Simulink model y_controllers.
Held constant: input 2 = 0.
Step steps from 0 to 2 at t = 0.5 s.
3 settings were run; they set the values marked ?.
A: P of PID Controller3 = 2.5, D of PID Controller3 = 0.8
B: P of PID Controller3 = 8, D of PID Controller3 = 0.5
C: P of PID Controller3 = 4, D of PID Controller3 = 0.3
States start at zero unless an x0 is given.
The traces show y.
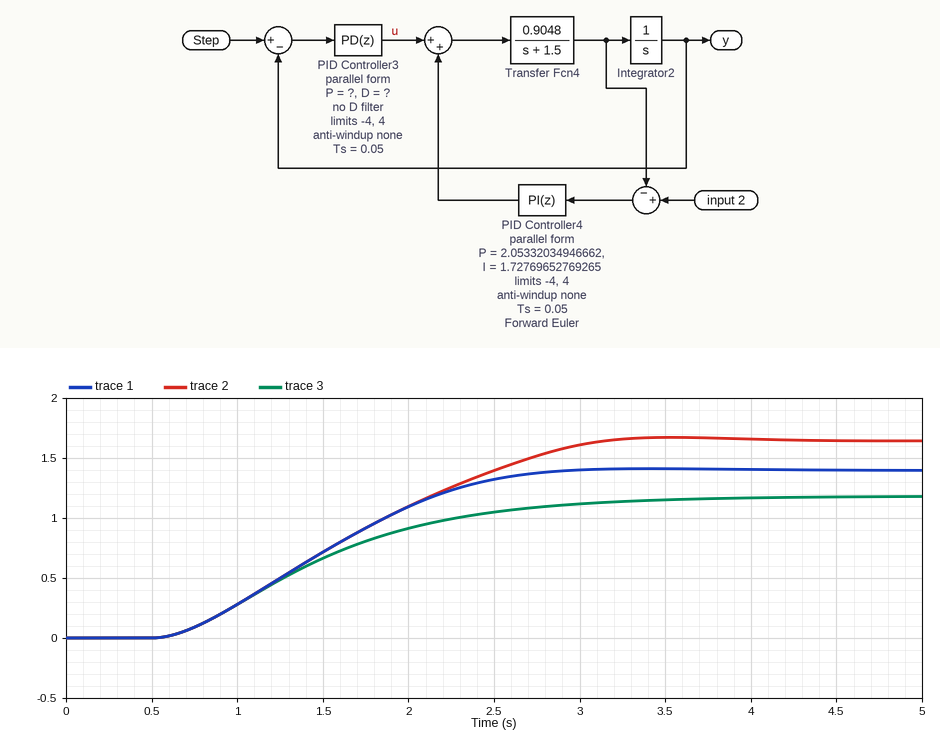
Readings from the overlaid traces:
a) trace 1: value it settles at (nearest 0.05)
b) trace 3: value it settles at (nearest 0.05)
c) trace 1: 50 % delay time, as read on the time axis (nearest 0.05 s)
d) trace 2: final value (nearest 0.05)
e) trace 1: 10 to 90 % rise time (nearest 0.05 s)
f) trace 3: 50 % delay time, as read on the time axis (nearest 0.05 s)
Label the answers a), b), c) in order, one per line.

a) 1.40
b) 1.20
c) 1.50 s
d) 1.65
e) 1.50 s
f) 1.40 s
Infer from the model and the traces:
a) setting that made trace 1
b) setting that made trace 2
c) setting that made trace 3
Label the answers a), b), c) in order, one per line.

a) C
b) B
c) A
